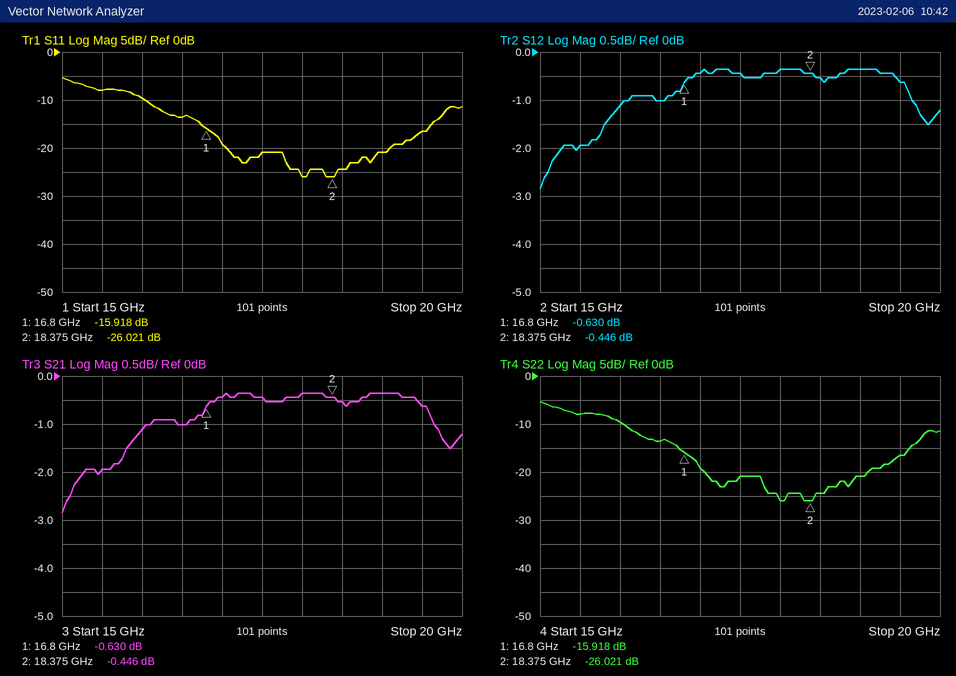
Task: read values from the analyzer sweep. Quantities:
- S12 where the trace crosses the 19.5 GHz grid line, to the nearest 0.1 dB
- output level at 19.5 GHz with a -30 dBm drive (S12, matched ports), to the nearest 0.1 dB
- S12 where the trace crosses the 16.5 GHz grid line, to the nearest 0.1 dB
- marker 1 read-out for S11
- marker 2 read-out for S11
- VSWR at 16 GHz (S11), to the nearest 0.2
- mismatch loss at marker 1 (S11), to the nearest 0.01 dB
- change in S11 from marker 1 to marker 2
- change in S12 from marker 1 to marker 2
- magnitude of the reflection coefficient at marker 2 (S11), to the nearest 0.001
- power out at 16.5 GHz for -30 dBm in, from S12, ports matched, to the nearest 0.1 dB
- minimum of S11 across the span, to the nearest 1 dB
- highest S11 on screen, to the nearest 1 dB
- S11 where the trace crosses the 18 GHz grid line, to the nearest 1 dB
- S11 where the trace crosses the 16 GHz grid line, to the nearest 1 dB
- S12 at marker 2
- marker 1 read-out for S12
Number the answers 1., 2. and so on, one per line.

1. -0.6 dB
2. -30.6 dBm
3. -1.0 dB
4. -15.918 dB
5. -26.021 dB
6. 2.0
7. 0.11 dB
8. -10.103 dB
9. 0.184 dB
10. 0.050
11. -31.0 dBm
12. -26 dB
13. -5 dB
14. -26 dB
15. -10 dB
16. -0.446 dB
17. -0.630 dB
